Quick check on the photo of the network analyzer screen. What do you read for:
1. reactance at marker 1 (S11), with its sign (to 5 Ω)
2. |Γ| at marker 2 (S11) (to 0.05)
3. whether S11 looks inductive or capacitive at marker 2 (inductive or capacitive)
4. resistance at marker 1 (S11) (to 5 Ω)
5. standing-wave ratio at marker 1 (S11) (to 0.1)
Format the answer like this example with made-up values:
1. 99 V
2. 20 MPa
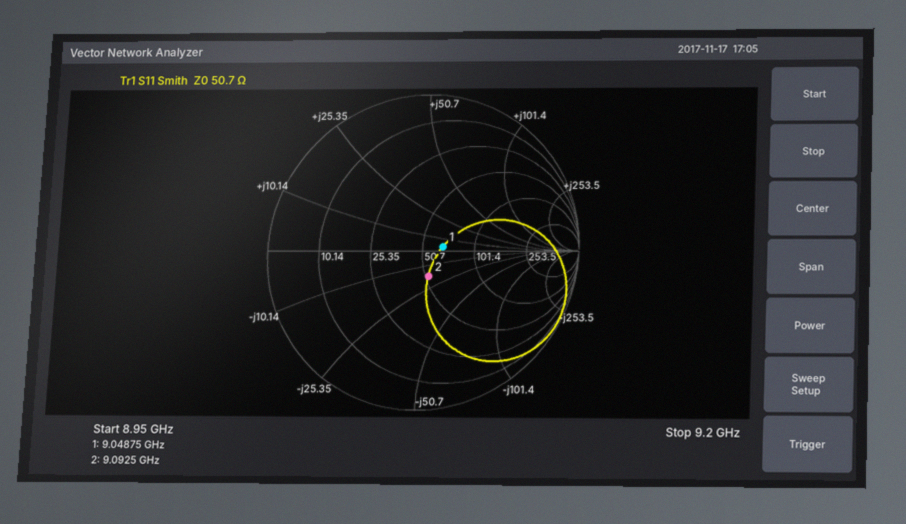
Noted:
1. +5 Ω
2. 0.15
3. capacitive
4. 65 Ω
5. 1.3
